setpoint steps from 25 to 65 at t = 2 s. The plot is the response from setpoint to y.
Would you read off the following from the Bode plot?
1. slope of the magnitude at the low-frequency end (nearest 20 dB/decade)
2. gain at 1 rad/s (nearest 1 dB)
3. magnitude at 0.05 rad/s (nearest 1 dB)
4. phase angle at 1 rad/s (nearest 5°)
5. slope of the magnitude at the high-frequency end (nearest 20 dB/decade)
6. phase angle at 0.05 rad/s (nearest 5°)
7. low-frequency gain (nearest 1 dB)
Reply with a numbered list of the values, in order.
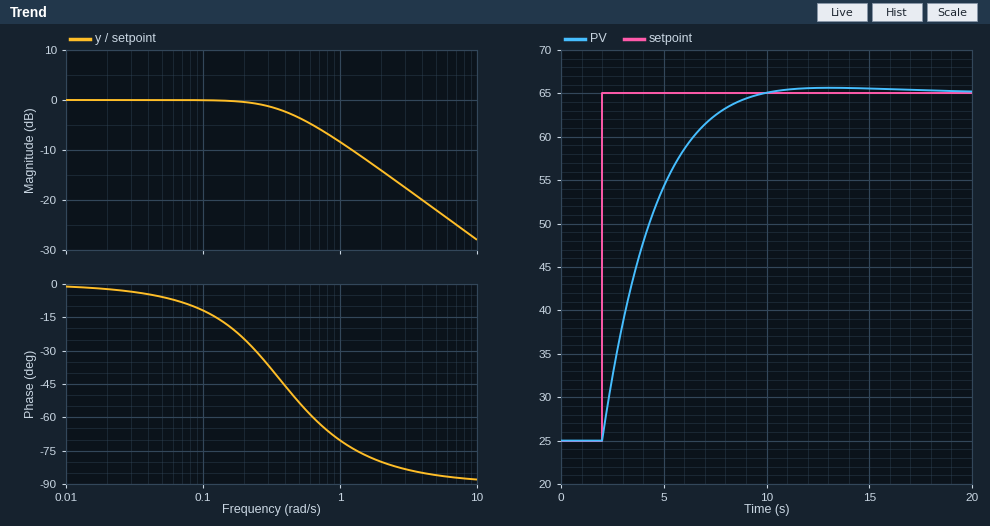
1. 0 dB/decade
2. -8 dB
3. 0 dB
4. -70°
5. -20 dB/decade
6. -5°
7. 0 dB
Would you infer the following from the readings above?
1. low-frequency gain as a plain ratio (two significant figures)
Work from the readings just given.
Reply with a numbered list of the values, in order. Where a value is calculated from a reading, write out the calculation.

1. 10^(0 / 20) = 1.0
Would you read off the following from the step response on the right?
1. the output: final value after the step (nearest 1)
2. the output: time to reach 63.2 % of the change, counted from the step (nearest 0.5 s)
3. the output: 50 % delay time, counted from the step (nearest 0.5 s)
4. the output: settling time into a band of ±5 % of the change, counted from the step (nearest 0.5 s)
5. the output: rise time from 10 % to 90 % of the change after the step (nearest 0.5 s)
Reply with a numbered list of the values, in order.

1. 65
2. 2.5 s
3. 1.5 s
4. 6.0 s
5. 4.5 s
